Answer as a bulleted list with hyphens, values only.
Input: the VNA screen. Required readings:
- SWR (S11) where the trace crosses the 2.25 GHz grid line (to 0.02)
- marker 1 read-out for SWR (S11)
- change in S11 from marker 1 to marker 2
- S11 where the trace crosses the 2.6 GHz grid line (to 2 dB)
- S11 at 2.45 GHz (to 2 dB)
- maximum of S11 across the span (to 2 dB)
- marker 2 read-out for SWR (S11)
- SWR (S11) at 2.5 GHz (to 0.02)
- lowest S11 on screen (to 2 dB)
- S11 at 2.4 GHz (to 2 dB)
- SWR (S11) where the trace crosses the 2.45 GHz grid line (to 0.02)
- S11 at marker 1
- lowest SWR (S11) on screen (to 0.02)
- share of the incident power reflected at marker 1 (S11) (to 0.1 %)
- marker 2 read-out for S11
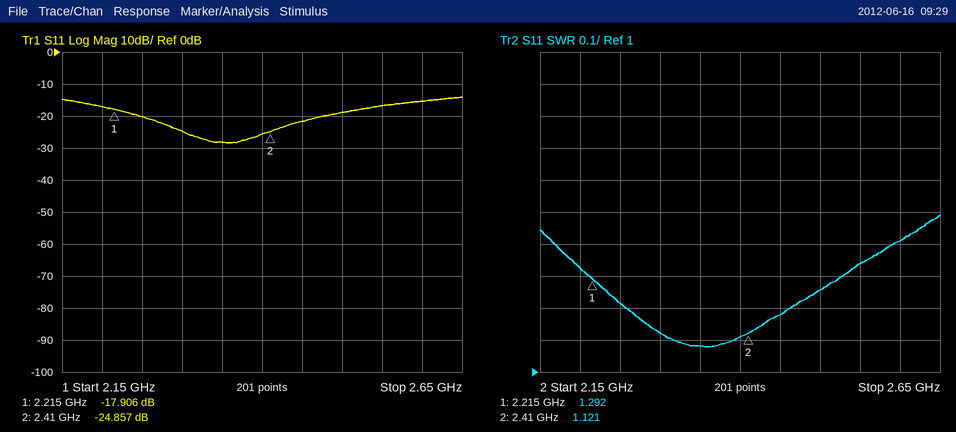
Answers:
- 1.22
- 1.292
- -6.951 dB
- -16 dB
- -22 dB
- -14 dB
- 1.121
- 1.26
- -28 dB
- -26 dB
- 1.18
- -17.906 dB
- 1.08
- 1.6 %
- -24.857 dB
